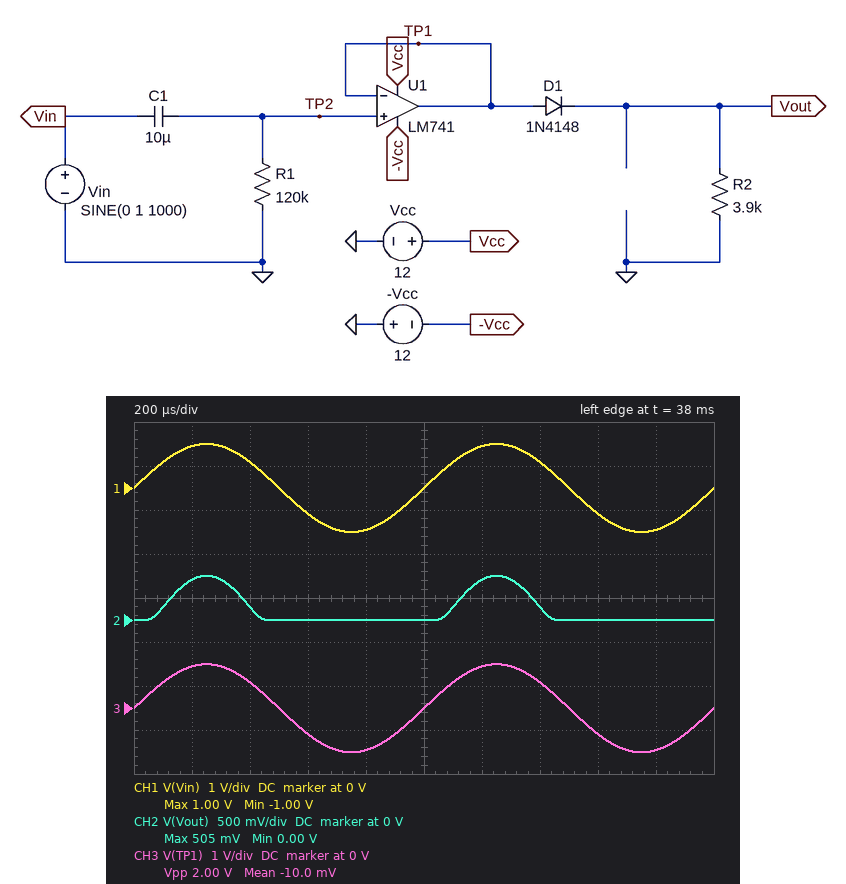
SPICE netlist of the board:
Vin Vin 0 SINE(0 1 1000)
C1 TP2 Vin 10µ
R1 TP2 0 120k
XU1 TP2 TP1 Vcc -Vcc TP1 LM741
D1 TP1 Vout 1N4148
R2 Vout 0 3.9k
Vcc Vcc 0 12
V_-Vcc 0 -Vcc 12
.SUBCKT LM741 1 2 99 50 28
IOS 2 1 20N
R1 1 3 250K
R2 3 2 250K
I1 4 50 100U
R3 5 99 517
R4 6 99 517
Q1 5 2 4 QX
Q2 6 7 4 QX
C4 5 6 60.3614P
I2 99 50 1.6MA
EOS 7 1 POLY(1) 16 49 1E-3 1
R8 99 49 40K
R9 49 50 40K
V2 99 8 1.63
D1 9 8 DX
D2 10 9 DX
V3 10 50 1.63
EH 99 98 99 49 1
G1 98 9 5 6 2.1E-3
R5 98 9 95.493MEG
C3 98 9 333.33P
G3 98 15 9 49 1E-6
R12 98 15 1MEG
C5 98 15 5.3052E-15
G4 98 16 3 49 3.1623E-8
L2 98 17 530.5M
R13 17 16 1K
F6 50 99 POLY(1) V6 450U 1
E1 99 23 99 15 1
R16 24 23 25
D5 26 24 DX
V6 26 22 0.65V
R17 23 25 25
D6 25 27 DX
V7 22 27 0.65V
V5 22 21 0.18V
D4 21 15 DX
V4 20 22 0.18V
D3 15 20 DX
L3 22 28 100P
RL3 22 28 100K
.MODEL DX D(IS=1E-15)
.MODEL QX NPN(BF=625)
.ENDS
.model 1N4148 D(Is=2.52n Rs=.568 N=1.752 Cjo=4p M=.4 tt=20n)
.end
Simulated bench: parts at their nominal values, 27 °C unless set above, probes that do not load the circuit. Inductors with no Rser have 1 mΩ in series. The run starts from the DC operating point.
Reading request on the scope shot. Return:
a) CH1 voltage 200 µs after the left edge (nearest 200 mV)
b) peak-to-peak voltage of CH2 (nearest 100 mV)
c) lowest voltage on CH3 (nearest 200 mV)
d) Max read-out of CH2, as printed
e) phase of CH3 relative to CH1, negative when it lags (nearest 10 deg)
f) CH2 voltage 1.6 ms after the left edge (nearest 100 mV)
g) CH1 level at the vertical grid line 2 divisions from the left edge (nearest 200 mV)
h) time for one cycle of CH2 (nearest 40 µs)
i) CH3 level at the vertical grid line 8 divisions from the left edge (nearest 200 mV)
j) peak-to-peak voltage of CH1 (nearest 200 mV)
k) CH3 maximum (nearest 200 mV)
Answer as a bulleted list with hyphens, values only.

- 1.0 V
- 500 mV
- -1.0 V
- 505 mV
- 0 deg
- 0 V
- 600 mV
- 1.00 ms
- -600 mV
- 2.0 V
- 1.0 V
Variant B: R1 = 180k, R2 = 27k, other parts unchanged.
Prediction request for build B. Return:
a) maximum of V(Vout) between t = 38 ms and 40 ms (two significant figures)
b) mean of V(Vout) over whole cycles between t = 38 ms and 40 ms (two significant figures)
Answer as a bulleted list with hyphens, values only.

- 580 mV
- 150 mV
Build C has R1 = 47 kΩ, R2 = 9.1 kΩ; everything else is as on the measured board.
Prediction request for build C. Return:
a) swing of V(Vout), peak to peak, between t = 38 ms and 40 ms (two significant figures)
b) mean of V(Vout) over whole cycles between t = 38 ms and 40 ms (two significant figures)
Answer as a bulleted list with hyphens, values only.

- 540 mV
- 130 mV
